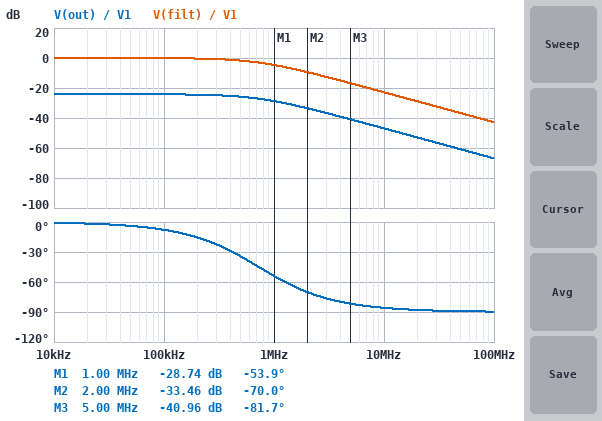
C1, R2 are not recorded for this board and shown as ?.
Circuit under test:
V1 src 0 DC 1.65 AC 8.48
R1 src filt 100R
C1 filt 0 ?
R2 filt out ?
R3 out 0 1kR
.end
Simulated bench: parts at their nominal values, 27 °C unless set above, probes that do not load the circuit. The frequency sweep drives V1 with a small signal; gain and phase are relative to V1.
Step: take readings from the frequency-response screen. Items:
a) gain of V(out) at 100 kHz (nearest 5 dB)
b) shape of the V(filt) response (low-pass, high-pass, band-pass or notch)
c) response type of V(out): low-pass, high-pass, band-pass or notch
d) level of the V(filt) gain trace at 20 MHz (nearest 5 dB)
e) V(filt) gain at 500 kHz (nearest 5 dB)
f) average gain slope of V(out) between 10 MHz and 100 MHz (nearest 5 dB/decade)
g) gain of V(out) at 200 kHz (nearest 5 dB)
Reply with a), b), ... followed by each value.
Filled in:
a) -25 dB
b) low-pass
c) low-pass
d) -30 dB
e) 0 dB
f) -20 dB/decade
g) -25 dB
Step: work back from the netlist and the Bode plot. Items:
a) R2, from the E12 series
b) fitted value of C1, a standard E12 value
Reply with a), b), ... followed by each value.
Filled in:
a) 15 kΩ
b) 2.2 nF
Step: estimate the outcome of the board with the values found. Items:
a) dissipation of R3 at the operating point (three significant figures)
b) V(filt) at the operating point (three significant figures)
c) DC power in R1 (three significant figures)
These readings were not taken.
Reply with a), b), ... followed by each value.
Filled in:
a) 10.5 µW
b) 1.64 V
c) 1.05 µW
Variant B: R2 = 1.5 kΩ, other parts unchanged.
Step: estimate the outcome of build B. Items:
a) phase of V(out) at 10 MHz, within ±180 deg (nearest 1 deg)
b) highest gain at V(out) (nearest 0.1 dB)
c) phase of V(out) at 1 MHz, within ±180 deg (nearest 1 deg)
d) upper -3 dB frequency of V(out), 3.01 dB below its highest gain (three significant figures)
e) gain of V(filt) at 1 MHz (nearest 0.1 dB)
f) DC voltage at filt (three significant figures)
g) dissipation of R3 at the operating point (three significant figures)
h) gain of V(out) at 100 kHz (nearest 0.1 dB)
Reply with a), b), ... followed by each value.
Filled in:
a) -86 deg
b) -8.3 dB
c) -53 deg
d) 752 kHz
e) -4.8 dB
f) 1.59 V
g) 403 µW
h) -8.4 dB
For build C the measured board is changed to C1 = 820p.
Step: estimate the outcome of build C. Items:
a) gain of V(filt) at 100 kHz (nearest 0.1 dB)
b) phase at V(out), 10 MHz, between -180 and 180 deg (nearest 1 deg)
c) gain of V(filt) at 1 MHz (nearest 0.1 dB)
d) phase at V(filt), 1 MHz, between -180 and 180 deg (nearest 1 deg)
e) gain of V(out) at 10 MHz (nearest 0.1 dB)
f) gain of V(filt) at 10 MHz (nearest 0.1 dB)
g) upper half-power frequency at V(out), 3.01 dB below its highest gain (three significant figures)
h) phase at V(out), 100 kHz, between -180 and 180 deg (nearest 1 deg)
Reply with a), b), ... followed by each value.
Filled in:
a) -0.1 dB
b) -79 deg
c) -1.1 dB
d) -27 deg
e) -38.5 dB
f) -14.4 dB
g) 1.95 MHz
h) -3 deg
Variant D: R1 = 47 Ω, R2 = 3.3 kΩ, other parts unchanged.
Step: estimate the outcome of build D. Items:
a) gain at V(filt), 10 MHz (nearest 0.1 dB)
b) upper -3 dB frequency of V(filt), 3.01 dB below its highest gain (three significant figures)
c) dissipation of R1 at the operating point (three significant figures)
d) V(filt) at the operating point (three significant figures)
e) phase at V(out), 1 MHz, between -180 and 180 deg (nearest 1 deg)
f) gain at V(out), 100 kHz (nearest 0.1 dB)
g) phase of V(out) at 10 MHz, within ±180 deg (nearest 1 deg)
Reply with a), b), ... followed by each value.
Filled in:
a) -16.4 dB
b) 1.56 MHz
c) 6.77 µW
d) 1.63 V
e) -33 deg
f) -12.8 dB
g) -81 deg
